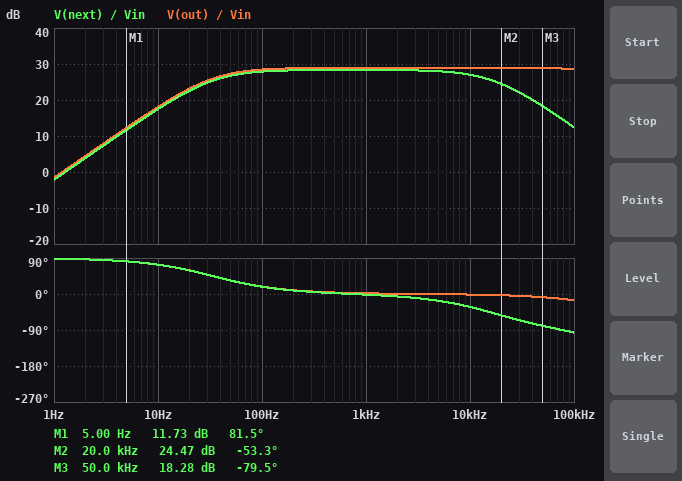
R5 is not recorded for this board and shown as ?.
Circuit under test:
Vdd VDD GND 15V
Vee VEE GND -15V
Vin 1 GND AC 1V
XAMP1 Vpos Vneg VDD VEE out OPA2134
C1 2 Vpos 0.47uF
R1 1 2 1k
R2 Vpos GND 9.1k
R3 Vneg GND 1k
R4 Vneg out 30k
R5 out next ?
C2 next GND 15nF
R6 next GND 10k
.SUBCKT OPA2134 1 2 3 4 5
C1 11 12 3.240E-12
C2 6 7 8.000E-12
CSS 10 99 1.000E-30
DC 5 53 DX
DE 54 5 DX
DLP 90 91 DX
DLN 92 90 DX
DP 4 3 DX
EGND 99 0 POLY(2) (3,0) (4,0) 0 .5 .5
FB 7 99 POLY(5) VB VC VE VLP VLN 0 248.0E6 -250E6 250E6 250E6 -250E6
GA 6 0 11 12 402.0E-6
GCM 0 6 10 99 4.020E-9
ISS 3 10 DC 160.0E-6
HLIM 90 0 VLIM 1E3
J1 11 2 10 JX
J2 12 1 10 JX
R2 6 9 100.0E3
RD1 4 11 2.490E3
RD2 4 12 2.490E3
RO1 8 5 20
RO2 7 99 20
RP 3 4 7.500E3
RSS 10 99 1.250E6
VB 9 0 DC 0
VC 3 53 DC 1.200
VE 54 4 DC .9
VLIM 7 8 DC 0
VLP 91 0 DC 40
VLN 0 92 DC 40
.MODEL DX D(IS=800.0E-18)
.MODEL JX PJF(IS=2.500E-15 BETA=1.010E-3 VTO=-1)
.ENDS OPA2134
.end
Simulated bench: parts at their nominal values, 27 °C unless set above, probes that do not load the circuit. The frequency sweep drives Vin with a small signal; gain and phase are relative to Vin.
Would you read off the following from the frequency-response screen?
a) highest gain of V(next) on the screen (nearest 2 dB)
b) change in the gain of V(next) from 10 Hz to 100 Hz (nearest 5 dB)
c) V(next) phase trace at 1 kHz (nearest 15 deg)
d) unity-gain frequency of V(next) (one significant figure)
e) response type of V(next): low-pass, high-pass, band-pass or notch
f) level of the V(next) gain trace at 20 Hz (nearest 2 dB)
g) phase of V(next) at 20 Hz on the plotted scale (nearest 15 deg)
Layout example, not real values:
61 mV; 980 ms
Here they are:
28 dB; 10 dB; 0 deg; 1 Hz; band-pass; 22 dB; 60 deg
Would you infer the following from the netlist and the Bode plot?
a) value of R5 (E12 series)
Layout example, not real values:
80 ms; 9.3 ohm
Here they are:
680 Ω
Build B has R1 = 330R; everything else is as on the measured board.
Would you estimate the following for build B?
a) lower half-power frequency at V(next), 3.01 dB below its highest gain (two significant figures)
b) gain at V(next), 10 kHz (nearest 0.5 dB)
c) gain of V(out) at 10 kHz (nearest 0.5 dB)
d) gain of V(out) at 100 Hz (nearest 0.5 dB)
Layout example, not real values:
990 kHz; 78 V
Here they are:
36 Hz; 27.5 dB; 29.5 dB; 29.0 dB
